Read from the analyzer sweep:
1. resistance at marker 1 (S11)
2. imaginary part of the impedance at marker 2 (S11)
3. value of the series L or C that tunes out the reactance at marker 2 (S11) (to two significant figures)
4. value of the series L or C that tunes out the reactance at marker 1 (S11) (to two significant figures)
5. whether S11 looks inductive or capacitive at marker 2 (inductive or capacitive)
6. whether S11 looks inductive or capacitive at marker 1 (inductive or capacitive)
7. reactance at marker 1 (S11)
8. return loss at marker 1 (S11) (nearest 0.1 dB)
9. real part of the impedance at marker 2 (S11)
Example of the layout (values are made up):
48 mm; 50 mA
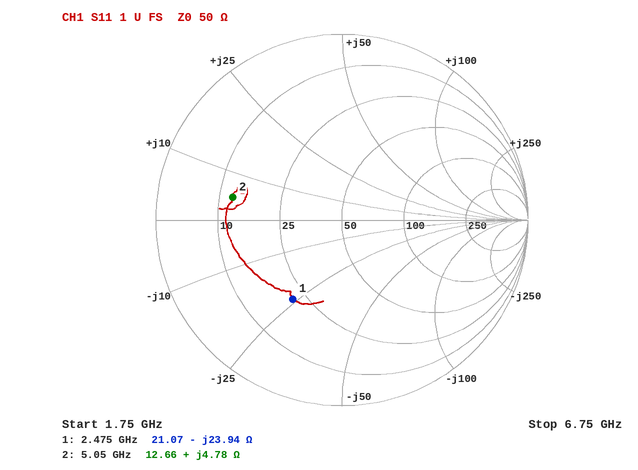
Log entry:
21.07 Ω; +4.78 Ω; 6.6 pF; 1.5 nH; inductive; capacitive; -23.94 Ω; 6.0 dB; 12.66 Ω
